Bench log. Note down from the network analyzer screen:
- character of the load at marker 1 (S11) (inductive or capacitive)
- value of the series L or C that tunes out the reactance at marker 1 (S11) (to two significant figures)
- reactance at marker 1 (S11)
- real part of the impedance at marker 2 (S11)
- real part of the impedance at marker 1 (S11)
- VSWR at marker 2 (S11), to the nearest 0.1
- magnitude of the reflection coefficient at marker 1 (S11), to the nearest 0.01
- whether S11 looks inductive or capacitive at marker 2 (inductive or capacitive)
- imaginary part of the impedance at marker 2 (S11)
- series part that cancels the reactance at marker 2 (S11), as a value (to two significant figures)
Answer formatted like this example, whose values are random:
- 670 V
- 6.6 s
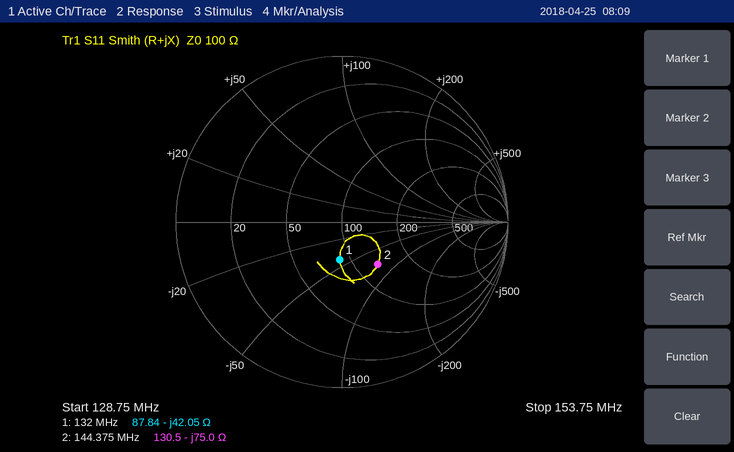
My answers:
- capacitive
- 51 nH
- -42.05 Ω
- 130.5 Ω
- 87.84 Ω
- 2.0
- 0.23
- capacitive
- -75.0 Ω
- 83 nH
